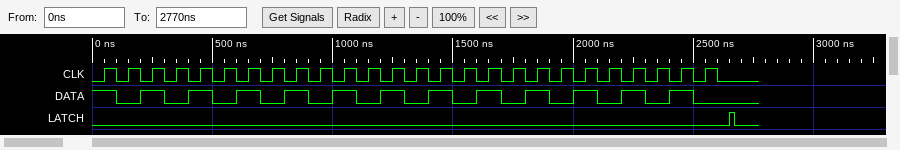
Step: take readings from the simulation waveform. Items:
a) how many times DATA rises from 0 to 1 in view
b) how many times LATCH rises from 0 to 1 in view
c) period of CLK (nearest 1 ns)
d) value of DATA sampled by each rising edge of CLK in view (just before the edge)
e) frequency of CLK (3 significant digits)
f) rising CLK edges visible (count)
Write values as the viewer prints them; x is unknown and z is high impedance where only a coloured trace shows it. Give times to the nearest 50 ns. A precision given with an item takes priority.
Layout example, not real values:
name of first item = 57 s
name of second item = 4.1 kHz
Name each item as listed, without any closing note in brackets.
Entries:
how many times DATA rises from 0 to 1 in view = 12
how many times LATCH rises from 0 to 1 in view = 1
period of CLK = 100 ns
value of DATA sampled by each rising edge of CLK in view = 1 0 1 0 1 0 1 0 1 0 1 0 1 0 1 0 1 0 1 0 1 0 1 0 1 0
frequency of CLK = 10.0 MHz
rising CLK edges visible = 26
